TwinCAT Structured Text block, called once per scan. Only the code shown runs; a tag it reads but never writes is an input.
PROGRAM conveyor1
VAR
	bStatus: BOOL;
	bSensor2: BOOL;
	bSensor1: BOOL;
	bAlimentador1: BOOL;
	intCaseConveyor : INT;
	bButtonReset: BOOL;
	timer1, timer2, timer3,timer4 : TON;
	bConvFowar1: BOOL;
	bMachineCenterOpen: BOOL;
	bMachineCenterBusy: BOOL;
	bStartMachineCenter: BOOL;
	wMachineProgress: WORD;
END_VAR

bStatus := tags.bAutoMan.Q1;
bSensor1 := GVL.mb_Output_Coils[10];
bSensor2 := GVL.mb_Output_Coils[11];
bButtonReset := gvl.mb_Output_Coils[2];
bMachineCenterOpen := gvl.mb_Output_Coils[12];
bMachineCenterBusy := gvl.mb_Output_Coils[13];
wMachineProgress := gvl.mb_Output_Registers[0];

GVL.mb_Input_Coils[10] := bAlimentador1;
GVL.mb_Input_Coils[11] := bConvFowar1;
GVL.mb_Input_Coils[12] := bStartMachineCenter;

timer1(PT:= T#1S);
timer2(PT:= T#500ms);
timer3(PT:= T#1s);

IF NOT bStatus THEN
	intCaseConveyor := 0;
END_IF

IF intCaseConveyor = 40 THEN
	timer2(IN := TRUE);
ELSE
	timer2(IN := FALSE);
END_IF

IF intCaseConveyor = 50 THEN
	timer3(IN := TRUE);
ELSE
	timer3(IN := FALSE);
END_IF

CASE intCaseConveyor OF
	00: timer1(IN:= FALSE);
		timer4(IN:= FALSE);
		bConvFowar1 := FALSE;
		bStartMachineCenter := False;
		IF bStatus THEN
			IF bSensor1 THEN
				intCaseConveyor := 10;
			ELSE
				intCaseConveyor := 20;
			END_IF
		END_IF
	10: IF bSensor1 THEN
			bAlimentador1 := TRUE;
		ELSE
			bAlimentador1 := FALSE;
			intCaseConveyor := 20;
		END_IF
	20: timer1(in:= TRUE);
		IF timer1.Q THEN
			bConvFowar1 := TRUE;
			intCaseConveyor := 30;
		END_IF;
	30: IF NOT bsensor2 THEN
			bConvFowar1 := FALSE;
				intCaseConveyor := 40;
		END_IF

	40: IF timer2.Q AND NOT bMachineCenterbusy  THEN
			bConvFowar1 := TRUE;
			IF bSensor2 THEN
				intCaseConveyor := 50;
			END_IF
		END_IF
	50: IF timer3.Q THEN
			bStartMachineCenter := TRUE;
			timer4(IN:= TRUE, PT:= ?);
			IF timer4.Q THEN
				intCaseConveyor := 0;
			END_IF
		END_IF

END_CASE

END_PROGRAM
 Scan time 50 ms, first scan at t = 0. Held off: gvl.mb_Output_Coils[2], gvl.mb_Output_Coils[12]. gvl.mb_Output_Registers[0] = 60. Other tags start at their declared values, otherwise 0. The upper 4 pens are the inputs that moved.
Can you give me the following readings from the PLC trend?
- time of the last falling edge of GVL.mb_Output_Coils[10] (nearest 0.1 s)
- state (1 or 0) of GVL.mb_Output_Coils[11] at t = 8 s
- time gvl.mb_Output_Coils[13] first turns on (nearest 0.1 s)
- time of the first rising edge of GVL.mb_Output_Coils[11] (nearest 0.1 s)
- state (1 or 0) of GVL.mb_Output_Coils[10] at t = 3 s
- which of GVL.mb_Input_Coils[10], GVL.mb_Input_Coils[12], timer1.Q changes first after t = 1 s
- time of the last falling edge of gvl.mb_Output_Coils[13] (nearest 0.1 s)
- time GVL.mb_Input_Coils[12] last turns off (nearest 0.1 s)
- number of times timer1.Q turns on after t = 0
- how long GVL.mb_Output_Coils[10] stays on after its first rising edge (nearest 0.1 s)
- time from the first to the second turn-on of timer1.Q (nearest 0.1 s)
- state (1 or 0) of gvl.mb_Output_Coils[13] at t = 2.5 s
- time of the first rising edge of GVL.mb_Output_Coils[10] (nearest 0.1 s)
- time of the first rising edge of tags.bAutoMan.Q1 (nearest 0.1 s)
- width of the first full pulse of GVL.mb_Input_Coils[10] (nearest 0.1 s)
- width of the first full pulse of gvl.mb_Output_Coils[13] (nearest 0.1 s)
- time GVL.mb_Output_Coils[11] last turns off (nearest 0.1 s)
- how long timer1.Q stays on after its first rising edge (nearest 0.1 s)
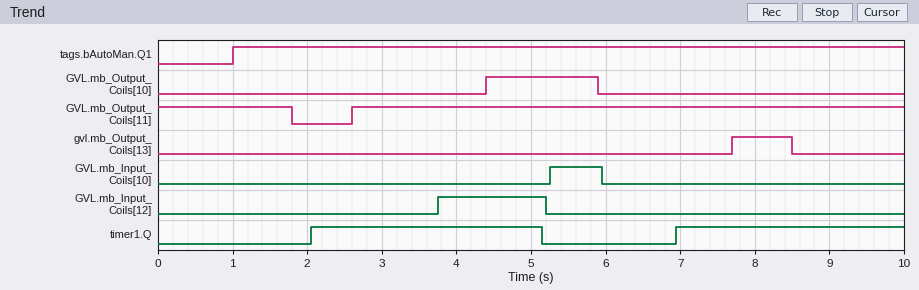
5.9 s
1
7.7 s
2.6 s
0
timer1.Q
8.5 s
5.2 s
2
1.5 s
4.9 s
0
4.4 s
1.0 s
0.7 s
0.8 s
1.8 s
3.1 s
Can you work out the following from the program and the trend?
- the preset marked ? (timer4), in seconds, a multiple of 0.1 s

1.4 s
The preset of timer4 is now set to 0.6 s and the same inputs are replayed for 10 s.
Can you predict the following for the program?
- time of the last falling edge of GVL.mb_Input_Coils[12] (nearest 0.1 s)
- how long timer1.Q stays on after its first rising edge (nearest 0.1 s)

4.4 s
2.3 s
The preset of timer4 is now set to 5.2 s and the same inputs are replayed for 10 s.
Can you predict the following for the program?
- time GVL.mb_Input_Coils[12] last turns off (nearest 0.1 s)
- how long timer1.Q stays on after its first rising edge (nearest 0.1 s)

9.0 s
6.9 s
